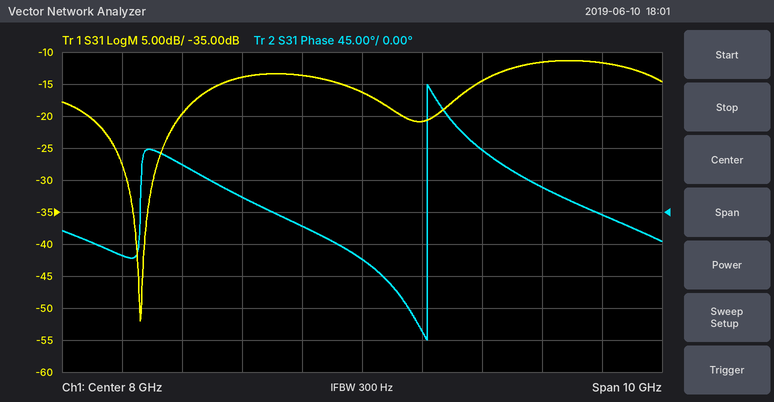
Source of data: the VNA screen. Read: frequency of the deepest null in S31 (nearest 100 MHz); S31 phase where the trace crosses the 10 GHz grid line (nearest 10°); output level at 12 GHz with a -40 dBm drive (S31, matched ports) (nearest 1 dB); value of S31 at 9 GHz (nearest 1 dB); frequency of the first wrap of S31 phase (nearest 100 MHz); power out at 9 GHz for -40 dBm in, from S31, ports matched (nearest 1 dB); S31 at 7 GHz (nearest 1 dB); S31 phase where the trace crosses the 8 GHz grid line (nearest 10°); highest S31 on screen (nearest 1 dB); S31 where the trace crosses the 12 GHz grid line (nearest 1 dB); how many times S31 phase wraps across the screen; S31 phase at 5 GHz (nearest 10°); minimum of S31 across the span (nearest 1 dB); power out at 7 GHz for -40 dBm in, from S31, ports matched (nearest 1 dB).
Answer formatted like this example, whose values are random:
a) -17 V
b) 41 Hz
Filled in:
a) 4.3 GHz
b) 90°
c) -52 dBm
d) -21 dB
e) 9.1 GHz
f) -61 dBm
g) -14 dB
h) -70°
i) -11 dB
j) -12 dB
k) 1
l) 70°
m) -52 dB
n) -54 dBm
